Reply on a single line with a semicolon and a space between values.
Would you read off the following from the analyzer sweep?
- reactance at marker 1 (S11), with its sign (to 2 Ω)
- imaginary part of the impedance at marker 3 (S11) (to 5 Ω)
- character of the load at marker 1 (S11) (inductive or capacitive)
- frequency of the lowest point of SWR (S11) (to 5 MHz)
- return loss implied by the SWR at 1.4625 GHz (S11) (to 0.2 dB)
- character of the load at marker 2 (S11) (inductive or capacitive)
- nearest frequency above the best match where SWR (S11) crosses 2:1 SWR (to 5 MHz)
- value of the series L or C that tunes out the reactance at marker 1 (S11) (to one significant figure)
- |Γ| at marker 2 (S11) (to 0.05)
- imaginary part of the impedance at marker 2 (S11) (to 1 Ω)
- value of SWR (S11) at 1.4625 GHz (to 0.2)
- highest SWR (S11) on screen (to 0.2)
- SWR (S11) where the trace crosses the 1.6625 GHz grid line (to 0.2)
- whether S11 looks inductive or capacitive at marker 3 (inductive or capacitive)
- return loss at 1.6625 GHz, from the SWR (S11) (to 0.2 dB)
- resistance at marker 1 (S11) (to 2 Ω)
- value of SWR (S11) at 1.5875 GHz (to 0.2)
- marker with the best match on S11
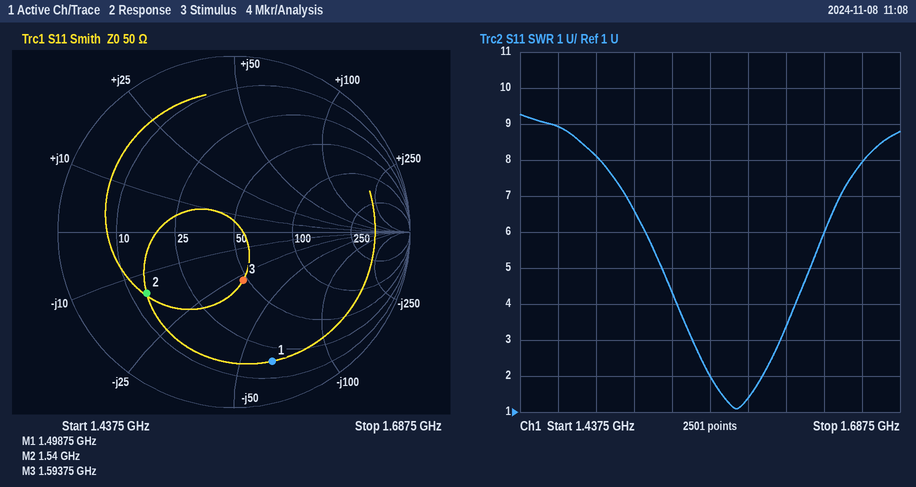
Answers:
-64 Ω; -30 Ω; capacitive; 1.580 GHz; 2.0 dB; capacitive; 1.595 GHz; 7 nH; 0.60; -15 Ω; 9.0; 9.2; 8.0; capacitive; 2.2 dB; 18 Ω; 1.4; marker 3
